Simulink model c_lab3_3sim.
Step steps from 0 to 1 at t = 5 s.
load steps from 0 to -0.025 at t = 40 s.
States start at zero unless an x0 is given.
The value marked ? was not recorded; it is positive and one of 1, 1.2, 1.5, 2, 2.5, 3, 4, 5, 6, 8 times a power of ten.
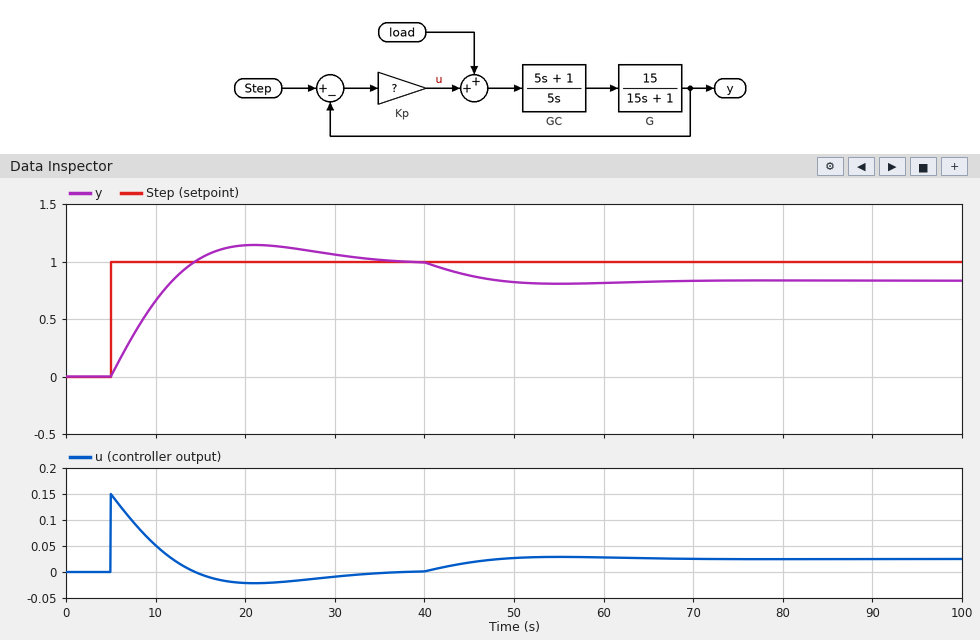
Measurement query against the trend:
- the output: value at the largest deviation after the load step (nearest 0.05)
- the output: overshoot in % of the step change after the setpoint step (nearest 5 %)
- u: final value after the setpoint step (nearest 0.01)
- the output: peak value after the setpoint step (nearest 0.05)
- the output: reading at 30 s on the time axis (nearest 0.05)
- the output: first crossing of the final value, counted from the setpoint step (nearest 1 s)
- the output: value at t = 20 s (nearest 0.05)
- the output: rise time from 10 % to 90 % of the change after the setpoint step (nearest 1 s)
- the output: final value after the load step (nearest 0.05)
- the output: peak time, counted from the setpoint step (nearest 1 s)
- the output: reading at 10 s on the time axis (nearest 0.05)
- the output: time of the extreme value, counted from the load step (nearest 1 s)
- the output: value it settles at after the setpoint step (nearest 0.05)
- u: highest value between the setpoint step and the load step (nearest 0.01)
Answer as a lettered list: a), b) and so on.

a) 0.80
b) 15 %
c) 0.00
d) 1.15
e) 1.05
f) 9 s
g) 1.15
h) 7 s
i) 0.85
j) 16 s
k) 0.65
l) 15 s
m) 1.00
n) 0.15
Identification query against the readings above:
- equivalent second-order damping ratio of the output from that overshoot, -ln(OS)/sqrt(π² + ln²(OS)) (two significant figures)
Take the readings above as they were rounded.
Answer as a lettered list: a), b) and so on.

a) 0.52
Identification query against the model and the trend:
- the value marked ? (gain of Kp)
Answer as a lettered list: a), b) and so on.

a) 0.15
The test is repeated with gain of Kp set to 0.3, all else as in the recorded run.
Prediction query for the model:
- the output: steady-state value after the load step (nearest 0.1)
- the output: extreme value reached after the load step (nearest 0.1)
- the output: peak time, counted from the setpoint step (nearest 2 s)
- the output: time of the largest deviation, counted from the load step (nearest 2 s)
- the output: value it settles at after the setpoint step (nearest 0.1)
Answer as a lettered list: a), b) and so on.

a) 0.9
b) 0.9
c) 10 s
d) 10 s
e) 1.0
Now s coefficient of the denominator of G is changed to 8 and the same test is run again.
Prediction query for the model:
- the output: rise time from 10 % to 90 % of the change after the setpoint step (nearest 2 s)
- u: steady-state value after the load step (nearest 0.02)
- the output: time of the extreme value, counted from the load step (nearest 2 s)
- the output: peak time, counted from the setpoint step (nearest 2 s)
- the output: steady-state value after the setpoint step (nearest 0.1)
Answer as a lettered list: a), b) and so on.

a) 6 s
b) 0.02
c) 12 s
d) 12 s
e) 1.0
